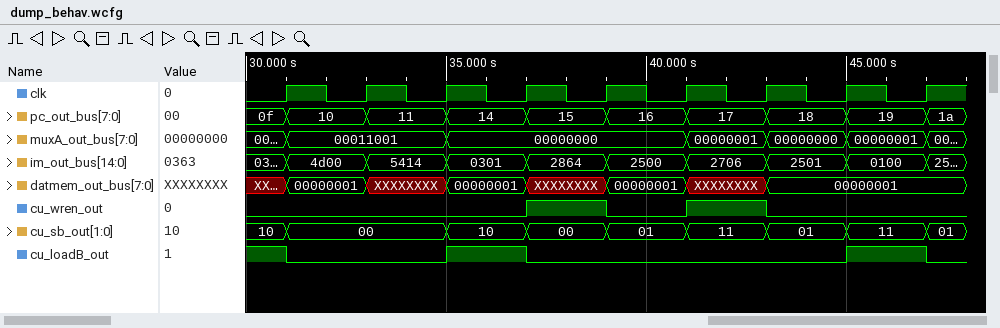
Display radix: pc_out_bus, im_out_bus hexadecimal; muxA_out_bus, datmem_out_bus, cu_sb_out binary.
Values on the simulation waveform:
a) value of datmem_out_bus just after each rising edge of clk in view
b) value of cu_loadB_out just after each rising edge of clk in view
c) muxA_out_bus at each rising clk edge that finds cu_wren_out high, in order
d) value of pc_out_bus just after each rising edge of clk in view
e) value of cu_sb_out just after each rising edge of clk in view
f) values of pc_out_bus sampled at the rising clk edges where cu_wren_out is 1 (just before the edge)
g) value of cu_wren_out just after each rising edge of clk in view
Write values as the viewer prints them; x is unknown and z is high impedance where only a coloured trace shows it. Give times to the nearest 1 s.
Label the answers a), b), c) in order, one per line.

a) 00000001, XXXXXXXX, 00000001, XXXXXXXX, 00000001, XXXXXXXX, 00000001, 00000001, 00000001
b) 0 0 1 0 0 0 0 1 0
c) 00000000, 00000001
d) 10, 11, 14, 15, 16, 17, 18, 19, 1a
e) 00, 00, 10, 00, 01, 11, 01, 11, 01
f) 15, 17
g) 0 0 0 1 0 1 0 0 0
